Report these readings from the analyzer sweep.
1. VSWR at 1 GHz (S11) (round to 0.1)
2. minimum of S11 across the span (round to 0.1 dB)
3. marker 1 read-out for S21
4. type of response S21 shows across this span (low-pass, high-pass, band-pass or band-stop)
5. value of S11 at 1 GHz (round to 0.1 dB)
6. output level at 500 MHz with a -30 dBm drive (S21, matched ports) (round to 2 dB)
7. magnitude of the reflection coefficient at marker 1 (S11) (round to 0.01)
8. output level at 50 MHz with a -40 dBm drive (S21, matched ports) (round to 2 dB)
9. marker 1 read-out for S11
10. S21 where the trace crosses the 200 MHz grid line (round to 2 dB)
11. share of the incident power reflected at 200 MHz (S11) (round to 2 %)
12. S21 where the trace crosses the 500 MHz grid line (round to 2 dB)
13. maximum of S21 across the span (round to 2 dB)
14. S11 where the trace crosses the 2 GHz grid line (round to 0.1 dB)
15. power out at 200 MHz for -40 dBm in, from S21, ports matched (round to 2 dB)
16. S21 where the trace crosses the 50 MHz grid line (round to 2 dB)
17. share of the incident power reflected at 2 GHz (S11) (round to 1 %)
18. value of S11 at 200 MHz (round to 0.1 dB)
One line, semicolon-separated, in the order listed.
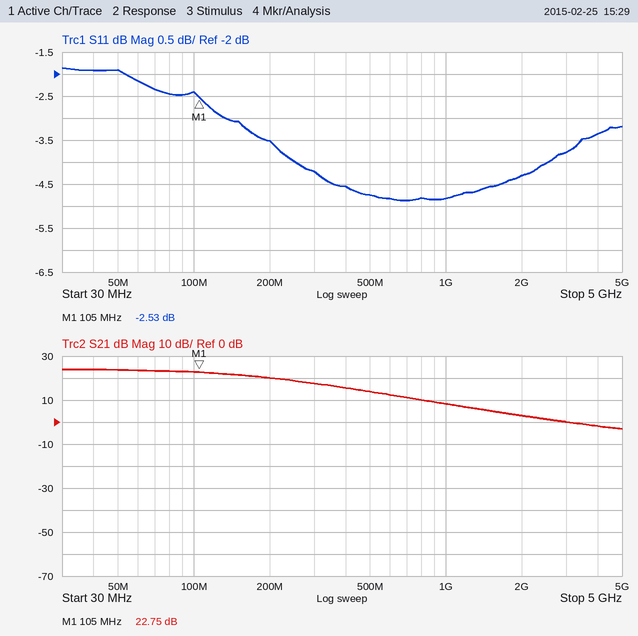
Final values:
3.7; -4.9 dB; 22.75 dB; low-pass; -4.8 dB; -16 dBm; 0.75; -16 dBm; -2.53 dB; 20 dB; 44 %; 14 dB; 24 dB; -4.3 dB; -20 dBm; 24 dB; 37 %; -3.5 dB
